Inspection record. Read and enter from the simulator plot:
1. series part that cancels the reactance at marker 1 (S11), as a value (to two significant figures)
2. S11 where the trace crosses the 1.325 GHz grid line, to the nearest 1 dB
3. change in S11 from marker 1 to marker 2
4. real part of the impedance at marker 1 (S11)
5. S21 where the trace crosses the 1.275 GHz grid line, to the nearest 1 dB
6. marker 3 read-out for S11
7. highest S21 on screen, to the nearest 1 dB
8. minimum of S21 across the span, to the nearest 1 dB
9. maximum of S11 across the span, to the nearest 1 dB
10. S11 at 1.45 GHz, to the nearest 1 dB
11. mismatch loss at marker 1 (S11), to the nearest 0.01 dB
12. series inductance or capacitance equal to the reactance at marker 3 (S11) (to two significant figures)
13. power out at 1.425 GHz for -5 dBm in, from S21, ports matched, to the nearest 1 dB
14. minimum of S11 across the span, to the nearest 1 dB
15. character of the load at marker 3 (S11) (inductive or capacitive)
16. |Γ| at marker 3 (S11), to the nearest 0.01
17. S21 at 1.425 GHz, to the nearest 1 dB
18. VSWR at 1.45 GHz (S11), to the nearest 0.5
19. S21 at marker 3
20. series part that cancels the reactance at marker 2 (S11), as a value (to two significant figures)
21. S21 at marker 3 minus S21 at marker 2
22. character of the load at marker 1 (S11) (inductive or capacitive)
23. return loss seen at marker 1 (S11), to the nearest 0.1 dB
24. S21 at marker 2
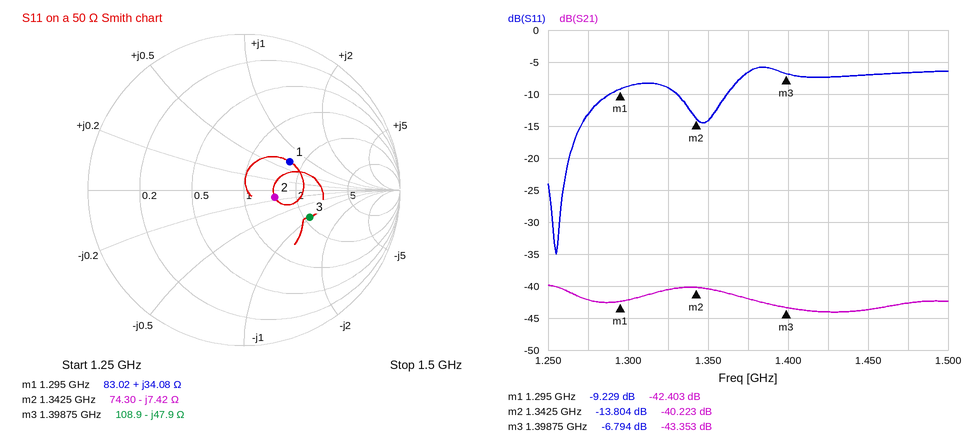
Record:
3.6 pF
-9 dB
-4.575 dB
83.02 Ω
-42 dB
-6.794 dB
-40 dB
-44 dB
-6 dB
-7 dB
0.55 dB
2.4 pF
-49 dBm
-35 dB
capacitive
0.46
-44 dB
2.5
-43.353 dB
880 pH
-3.130 dB
inductive
9.2 dB
-40.223 dB
